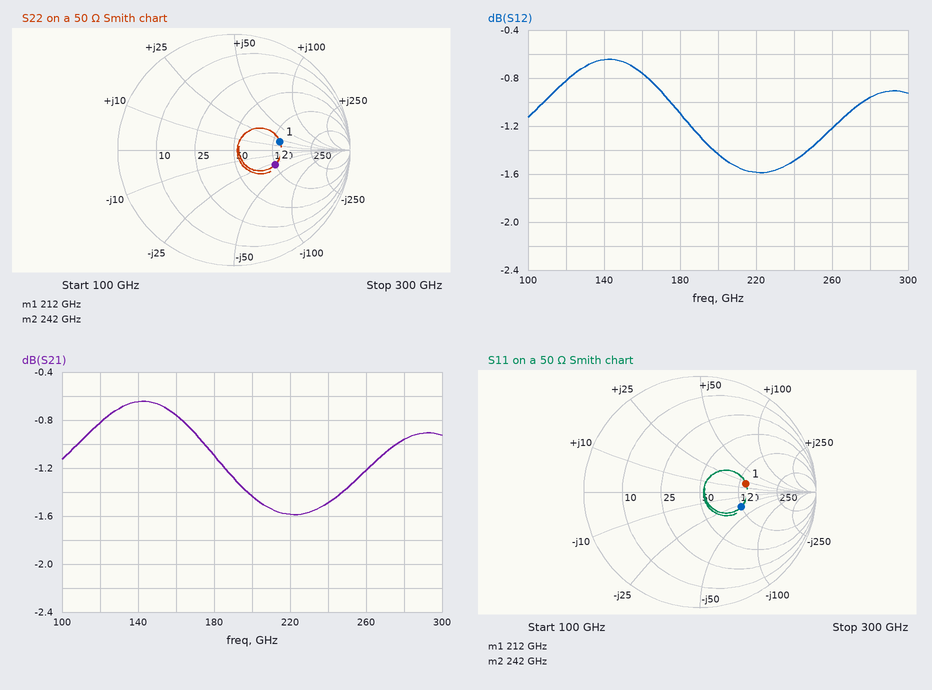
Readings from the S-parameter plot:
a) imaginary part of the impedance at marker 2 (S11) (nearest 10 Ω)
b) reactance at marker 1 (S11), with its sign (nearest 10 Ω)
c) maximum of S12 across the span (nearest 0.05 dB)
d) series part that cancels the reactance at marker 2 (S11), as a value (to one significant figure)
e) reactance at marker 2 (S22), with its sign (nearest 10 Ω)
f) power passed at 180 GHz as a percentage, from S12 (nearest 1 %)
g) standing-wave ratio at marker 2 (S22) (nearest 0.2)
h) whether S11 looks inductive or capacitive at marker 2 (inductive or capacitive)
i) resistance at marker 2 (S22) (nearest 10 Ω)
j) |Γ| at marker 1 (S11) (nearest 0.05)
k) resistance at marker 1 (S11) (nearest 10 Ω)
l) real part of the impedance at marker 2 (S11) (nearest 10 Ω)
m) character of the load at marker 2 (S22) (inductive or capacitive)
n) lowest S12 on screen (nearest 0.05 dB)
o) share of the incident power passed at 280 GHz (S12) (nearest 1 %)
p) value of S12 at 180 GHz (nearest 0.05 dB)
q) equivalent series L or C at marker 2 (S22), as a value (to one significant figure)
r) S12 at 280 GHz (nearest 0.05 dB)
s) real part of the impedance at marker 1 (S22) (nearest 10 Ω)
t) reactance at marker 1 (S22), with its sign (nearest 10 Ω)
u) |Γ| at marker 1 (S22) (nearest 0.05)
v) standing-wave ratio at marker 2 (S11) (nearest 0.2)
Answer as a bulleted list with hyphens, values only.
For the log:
- -30 Ω
- +20 Ω
- -0.65 dB
- 20 pH
- -30 Ω
- 78 %
- 2.2
- capacitive
- 100 Ω
- 0.40
- 110 Ω
- 100 Ω
- capacitive
- -1.60 dB
- 80 %
- -1.10 dB
- 20 fF
- -0.95 dB
- 110 Ω
- +20 Ω
- 0.40
- 2.2
